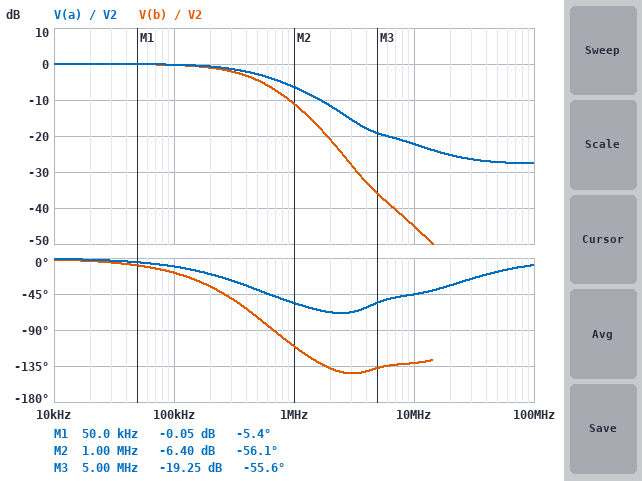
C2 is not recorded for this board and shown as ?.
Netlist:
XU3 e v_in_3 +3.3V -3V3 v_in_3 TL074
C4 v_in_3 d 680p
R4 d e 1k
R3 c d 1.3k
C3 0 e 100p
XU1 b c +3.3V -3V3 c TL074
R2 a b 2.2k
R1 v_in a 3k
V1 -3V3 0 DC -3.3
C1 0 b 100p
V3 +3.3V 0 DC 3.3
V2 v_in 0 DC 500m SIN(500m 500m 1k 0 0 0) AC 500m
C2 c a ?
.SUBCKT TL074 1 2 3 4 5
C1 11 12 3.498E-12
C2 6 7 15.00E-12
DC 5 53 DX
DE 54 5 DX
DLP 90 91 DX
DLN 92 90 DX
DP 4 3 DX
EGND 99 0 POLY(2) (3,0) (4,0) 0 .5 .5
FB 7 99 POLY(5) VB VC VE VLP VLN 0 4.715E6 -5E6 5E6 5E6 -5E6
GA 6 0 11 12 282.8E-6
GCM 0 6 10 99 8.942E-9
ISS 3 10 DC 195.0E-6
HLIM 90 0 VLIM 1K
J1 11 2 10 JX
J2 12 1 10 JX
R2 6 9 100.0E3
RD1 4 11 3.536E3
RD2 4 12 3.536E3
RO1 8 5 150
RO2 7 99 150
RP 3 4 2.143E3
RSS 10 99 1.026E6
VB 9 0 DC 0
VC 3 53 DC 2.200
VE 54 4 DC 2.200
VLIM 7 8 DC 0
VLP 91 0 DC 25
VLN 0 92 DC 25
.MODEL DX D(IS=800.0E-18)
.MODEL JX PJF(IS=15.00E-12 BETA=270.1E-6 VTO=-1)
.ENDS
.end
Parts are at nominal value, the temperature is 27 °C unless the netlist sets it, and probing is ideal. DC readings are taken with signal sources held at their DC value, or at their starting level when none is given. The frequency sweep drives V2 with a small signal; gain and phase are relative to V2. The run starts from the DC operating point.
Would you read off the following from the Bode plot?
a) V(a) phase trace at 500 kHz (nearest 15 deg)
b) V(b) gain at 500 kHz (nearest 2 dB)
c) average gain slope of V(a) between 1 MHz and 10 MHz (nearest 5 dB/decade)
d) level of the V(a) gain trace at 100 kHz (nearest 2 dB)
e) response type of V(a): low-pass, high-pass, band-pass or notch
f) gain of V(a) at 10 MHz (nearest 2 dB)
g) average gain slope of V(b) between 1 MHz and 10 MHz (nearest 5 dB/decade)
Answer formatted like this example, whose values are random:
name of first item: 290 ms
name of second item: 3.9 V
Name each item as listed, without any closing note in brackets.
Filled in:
V(a) phase trace at 500 kHz: -45 deg
V(b) gain at 500 kHz: -4 dB
average gain slope of V(a) between 1 MHz and 10 MHz: -15 dB/decade
level of the V(a) gain trace at 100 kHz: 0 dB
response type of V(a): low-pass, high-pass, band-pass or notch: low-pass
gain of V(a) at 10 MHz: -22 dB
average gain slope of V(b) between 1 MHz and 10 MHz: -35 dB/decade
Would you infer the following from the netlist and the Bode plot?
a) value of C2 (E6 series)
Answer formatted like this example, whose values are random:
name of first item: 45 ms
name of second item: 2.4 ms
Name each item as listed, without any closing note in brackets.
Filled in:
value of C2: 68 pF
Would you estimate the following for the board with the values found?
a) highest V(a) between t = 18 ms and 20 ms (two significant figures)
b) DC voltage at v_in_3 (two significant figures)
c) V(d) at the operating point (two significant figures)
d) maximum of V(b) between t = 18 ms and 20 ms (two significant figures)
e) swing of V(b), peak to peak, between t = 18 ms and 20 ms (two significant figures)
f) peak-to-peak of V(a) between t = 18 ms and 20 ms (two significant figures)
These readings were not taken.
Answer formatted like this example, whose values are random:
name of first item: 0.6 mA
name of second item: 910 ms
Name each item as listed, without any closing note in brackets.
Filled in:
highest V(a) between t = 18 ms and 20 ms: 1.0 V
DC voltage at v_in_3: 500 mV
V(d) at the operating point: 500 mV
maximum of V(b) between t = 18 ms and 20 ms: 1.0 V
swing of V(b), peak to peak, between t = 18 ms and 20 ms: 1.0 V
peak-to-peak of V(a) between t = 18 ms and 20 ms: 1.0 V
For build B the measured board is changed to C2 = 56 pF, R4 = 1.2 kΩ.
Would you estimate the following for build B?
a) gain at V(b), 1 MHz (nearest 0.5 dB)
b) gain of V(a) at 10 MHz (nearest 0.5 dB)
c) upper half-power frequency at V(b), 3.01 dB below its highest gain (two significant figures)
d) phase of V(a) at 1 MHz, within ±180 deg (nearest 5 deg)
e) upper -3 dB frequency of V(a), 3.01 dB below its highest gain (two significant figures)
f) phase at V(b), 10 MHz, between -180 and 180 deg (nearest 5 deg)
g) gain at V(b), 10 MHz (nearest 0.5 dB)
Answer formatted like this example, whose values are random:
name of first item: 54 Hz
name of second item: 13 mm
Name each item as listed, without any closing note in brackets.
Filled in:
gain at V(b), 1 MHz: -10.5 dB
gain of V(a) at 10 MHz: -21.0 dB
upper half-power frequency at V(b), 3.01 dB below its highest gain: 370 kHz
phase of V(a) at 1 MHz, within ±180 deg: -50 deg
upper -3 dB frequency of V(a), 3.01 dB below its highest gain: 500 kHz
phase at V(b), 10 MHz, between -180 and 180 deg: -135 deg
gain at V(b), 10 MHz: -44.0 dB
